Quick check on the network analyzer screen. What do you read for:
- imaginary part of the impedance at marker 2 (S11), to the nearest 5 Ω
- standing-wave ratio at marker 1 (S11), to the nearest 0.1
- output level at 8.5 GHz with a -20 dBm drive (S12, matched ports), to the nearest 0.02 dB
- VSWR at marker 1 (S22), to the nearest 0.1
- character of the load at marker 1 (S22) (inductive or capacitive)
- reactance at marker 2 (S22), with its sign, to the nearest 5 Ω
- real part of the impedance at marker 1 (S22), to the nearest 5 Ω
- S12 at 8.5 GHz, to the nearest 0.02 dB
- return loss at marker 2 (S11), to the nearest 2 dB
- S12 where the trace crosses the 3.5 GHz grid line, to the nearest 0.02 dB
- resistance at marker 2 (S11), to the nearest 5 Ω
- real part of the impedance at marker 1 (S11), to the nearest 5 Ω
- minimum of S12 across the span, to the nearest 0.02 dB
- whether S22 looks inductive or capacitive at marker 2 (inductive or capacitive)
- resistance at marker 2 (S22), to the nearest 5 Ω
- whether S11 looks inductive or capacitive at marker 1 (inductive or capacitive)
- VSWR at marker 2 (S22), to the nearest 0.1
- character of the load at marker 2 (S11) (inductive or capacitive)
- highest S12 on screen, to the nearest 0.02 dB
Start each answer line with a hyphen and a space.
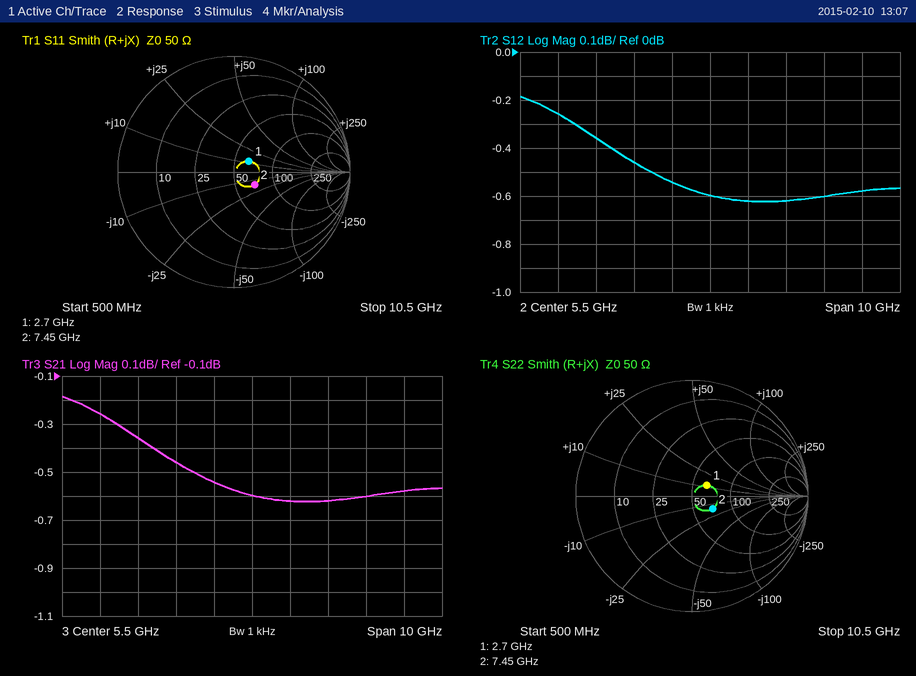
- -15 Ω
- 1.4
- -20.60 dBm
- 1.4
- inductive
- -15 Ω
- 65 Ω
- -0.60 dB
- 14 dB
- -0.46 dB
- 70 Ω
- 65 Ω
- -0.62 dB
- capacitive
- 70 Ω
- inductive
- 1.5
- capacitive
- -0.18 dB
